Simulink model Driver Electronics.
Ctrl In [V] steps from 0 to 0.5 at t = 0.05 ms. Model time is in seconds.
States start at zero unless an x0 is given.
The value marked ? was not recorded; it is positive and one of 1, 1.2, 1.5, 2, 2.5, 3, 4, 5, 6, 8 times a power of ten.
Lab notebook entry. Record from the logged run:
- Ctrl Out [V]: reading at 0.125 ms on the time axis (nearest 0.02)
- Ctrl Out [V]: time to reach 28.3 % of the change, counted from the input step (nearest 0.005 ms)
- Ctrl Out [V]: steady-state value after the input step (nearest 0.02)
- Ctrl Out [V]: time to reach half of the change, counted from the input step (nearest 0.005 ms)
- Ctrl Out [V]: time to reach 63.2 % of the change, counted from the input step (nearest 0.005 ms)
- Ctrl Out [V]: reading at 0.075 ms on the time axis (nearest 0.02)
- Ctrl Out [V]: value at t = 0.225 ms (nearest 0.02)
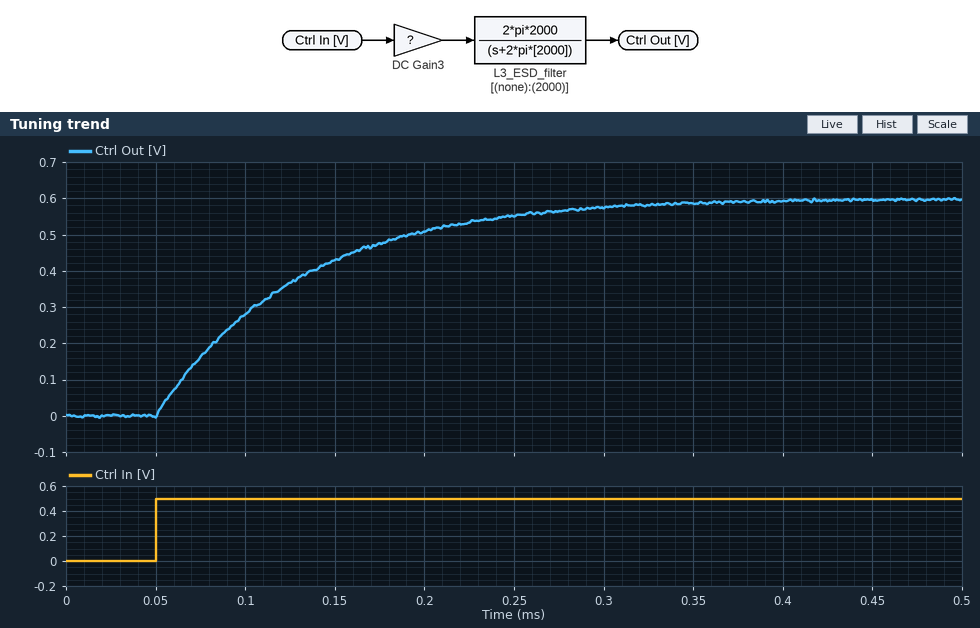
0.36
0.025 ms
0.60
0.055 ms
0.080 ms
0.16
0.54
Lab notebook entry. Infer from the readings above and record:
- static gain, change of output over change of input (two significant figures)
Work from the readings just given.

1.2
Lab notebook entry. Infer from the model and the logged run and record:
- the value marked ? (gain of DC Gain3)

1.2
